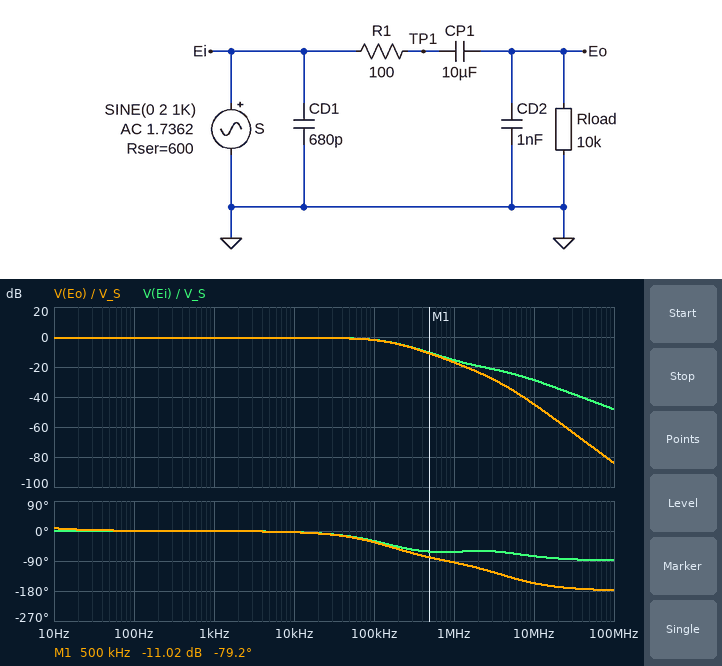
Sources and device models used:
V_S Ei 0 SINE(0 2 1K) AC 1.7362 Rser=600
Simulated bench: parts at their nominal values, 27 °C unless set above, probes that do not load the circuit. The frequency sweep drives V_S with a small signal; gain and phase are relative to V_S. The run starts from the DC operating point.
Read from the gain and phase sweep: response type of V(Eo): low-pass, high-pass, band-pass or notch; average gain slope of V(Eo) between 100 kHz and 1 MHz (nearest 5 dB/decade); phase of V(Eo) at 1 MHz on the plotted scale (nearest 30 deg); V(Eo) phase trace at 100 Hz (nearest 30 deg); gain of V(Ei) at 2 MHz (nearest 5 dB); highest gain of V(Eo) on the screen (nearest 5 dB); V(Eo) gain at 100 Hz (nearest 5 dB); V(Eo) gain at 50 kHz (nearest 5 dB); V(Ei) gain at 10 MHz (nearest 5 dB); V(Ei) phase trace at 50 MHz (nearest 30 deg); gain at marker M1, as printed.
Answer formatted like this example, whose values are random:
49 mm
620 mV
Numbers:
low-pass
-15 dB/decade
-90 deg
0 deg
-20 dB
0 dB
0 dB
0 dB
-30 dB
-90 deg
-11.02 dB
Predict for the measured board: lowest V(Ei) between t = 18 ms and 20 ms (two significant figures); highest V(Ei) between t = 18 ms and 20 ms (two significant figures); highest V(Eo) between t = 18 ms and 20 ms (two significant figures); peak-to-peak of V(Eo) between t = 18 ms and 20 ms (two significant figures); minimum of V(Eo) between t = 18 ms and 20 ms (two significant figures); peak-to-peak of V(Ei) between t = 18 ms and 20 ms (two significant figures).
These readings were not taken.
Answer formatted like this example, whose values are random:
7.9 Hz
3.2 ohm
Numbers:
-1.9 V
1.9 V
1.9 V
3.7 V
-1.9 V
3.8 V
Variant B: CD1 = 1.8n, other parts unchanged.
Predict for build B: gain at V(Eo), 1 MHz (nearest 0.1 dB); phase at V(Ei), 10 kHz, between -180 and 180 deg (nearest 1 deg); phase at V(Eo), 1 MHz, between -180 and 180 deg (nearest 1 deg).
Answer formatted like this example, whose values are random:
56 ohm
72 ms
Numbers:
-21.4 dB
-6 deg
-106 deg
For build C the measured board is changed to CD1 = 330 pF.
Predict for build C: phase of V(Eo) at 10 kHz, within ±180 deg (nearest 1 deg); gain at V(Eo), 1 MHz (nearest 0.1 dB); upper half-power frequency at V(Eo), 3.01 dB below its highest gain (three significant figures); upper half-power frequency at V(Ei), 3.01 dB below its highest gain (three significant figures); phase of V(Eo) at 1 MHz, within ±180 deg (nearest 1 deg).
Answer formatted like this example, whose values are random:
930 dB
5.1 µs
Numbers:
-3 deg
-15.1 dB
194 kHz
174 kHz
-87 deg
